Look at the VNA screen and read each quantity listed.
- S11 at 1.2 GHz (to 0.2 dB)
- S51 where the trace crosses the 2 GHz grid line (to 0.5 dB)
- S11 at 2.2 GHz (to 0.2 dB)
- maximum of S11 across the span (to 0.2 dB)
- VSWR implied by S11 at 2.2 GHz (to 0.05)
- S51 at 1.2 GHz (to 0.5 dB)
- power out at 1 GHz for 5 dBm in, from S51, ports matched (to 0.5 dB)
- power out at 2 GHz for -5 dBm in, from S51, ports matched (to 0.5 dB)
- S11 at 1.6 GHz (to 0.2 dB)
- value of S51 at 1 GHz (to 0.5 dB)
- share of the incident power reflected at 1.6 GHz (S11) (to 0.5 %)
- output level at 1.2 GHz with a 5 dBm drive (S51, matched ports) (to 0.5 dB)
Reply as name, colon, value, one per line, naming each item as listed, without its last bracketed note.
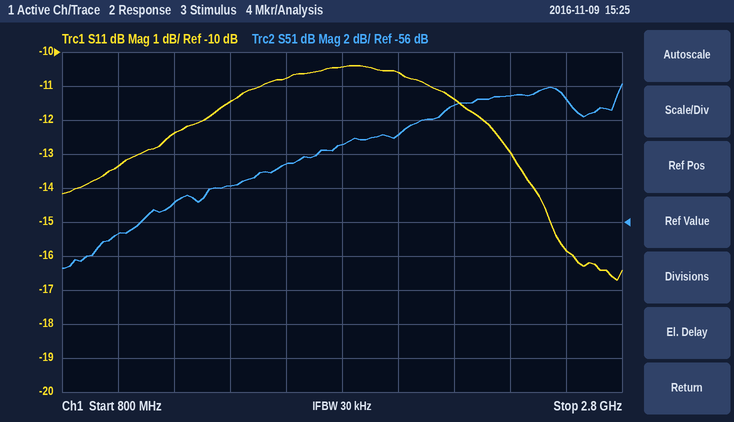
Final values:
S11 at 1.2 GHz: -12.4 dB
S51 where the trace crosses the 2 GHz grid line: -51.0 dB
S11 at 2.2 GHz: -11.4 dB
maximum of S11 across the span: -10.4 dB
VSWR implied by S11 at 2.2 GHz: 1.75
S51 at 1.2 GHz: -55.0 dB
power out at 1 GHz for 5 dBm in, from S51, ports matched: -51.5 dBm
power out at 2 GHz for -5 dBm in, from S51, ports matched: -56.0 dBm
S11 at 1.6 GHz: -10.8 dB
value of S51 at 1 GHz: -56.5 dB
share of the incident power reflected at 1.6 GHz (S11): 8.5 %
output level at 1.2 GHz with a 5 dBm drive (S51, matched ports): -50.0 dBm
